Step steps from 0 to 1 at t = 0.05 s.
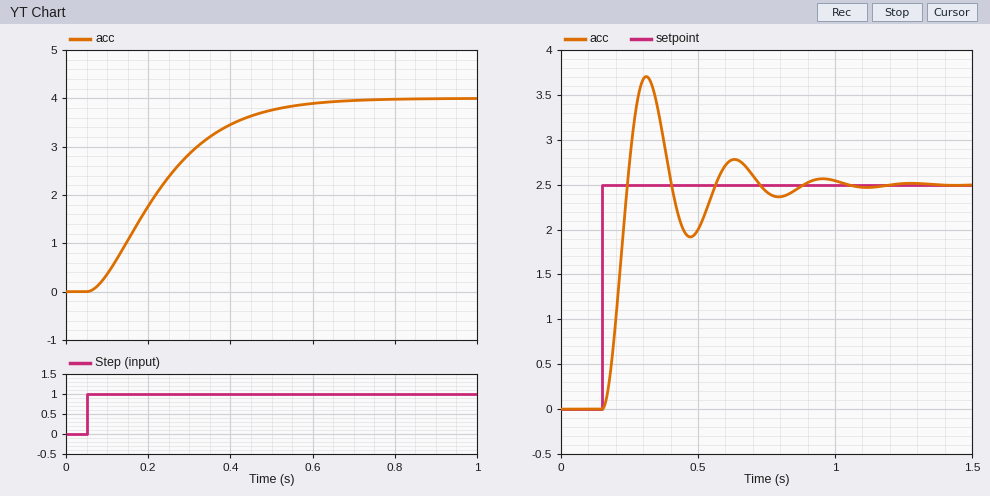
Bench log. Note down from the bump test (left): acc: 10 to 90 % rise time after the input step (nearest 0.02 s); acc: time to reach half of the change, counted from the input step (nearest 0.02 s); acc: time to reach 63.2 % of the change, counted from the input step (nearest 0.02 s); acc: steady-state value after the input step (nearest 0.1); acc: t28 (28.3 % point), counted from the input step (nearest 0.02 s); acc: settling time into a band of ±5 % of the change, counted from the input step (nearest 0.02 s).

0.34 s
0.16 s
0.22 s
4.0
0.10 s
0.48 s
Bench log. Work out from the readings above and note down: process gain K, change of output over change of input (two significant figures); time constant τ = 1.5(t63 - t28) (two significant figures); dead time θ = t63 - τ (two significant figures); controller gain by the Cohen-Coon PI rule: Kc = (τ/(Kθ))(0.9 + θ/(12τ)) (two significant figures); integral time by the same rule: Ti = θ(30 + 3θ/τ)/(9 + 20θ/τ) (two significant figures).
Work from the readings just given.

4.0
0.18 s
0.040 s
1.0
0.091 s
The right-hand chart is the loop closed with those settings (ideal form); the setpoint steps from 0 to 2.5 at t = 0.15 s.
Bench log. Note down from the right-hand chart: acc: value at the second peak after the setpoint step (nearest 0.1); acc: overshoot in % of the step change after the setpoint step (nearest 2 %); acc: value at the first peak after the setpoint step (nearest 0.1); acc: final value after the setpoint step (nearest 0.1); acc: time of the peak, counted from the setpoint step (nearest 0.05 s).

2.8
48 %
3.7
2.5
0.15 s
